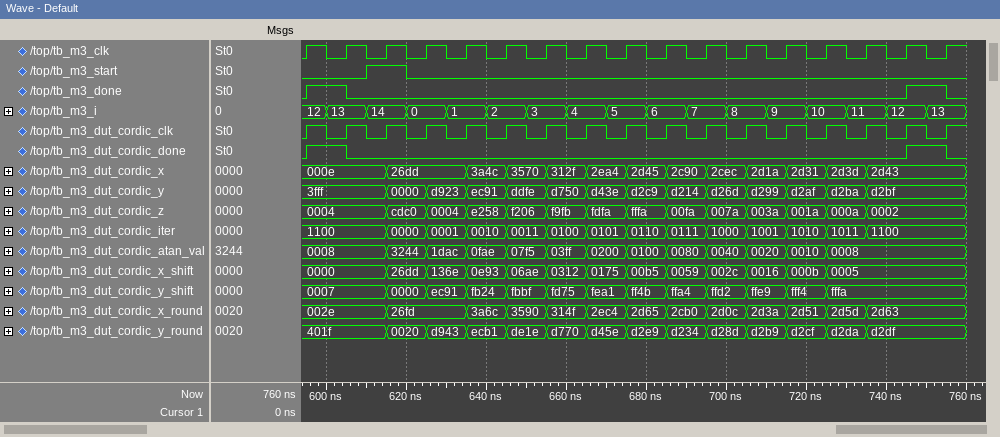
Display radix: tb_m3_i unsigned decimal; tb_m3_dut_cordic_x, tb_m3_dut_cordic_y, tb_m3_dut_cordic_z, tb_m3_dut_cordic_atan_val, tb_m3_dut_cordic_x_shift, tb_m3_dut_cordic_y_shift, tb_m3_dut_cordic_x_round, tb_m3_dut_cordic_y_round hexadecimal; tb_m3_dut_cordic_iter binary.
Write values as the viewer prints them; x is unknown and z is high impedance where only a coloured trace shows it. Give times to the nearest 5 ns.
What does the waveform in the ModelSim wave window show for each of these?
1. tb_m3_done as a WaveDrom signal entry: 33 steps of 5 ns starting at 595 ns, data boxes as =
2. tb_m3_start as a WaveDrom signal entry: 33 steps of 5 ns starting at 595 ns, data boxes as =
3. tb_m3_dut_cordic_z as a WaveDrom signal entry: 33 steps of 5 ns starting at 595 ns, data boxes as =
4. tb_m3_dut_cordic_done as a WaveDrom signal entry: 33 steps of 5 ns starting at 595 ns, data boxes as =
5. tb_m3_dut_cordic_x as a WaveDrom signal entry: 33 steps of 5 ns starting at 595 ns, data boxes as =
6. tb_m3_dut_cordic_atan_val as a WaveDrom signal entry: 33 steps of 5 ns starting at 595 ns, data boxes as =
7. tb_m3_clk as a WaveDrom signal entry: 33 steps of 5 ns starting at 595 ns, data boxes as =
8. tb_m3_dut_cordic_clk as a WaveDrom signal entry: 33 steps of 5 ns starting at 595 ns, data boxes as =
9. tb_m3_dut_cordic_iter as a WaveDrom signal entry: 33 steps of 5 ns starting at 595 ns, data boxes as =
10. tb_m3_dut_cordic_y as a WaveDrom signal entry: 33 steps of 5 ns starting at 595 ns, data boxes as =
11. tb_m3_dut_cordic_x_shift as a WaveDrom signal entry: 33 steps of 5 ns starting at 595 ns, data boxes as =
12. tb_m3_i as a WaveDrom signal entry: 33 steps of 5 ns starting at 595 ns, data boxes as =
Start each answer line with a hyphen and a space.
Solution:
- {name: 'tb_m3_done', wave: '1.0...........................1.0'}
- {name: 'tb_m3_start', wave: '0..1.0...........................'}
- {name: 'tb_m3_dut_cordic_z', wave: '=...=.=.=.=.=.=.=.=.=.=.=.=.=....', data: '0004 cdc0 0004 e258 f206 f9fb fdfa fffa 00fa 007a 003a 001a 000a 0002'}
- {name: 'tb_m3_dut_cordic_done', wave: '1.0...........................1.0'}
- {name: 'tb_m3_dut_cordic_x', wave: '=...=...=.=.=.=.=.=.=.=.=.=.=....', data: '000e 26dd 3a4c 3570 312f 2ea4 2d45 2c90 2cec 2d1a 2d31 2d3d 2d43'}
- {name: 'tb_m3_dut_cordic_atan_val', wave: '=...=.=.=.=.=.=.=.=.=.=.=.=......', data: '0008 3244 1dac 0fae 07f5 03ff 0200 0100 0080 0040 0020 0010 0008'}
- {name: 'tb_m3_clk', wave: '101010101010101010101010101010101'}
- {name: 'tb_m3_dut_cordic_clk', wave: '101010101010101010101010101010101'}
- {name: 'tb_m3_dut_cordic_iter', wave: '=...=.=.=.=.=.=.=.=.=.=.=.=.=....', data: '1100 0000 0001 0010 0011 0100 0101 0110 0111 1000 1001 1010 1011 1100'}
- {name: 'tb_m3_dut_cordic_y', wave: '=...=.=.=.=.=.=.=.=.=.=.=.=.=....', data: '3fff 0000 d923 ec91 ddfe d750 d43e d2c9 d214 d26d d299 d2af d2ba d2bf'}
- {name: 'tb_m3_dut_cordic_x_shift', wave: '=...=.=.=.=.=.=.=.=.=.=.=.=......', data: '0000 26dd 136e 0e93 06ae 0312 0175 00b5 0059 002c 0016 000b 0005'}
- {name: 'tb_m3_i', wave: '==.=.=.=.=.=.=.=.=.=.=.=.=.=.=.=.', data: '12 13 14 0 1 2 3 4 5 6 7 8 9 10 11 12 13'}
